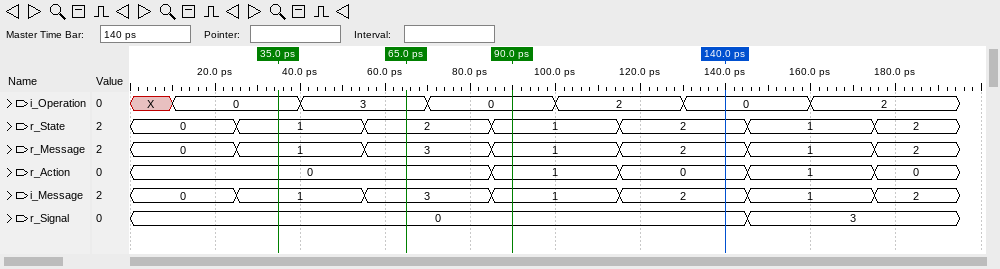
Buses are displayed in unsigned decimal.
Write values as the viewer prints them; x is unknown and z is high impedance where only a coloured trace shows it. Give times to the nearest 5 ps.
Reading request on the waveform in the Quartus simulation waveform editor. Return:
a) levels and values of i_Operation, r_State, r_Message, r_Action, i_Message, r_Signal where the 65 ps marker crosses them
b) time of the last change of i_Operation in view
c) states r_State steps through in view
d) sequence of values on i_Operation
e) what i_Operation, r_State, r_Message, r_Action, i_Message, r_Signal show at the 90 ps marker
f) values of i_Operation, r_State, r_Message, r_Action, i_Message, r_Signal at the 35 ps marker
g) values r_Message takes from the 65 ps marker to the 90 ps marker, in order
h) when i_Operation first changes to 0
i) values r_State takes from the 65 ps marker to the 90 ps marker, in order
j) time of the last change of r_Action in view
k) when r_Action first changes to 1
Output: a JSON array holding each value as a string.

["i_Operation=3, r_State=2, r_Message=3, r_Action=0, i_Message=3, r_Signal=0", "160 ps", "0, 1, 2, 1, 2, 1, 2", "X, 0, 3, 0, 2, 0, 2", "i_Operation=0, r_State=1, r_Message=1, r_Action=1, i_Message=1, r_Signal=0", "i_Operation=0, r_State=1, r_Message=1, r_Action=0, i_Message=1, r_Signal=0", "3, 1", "10 ps", "2, 1", "175 ps", "85 ps"]
